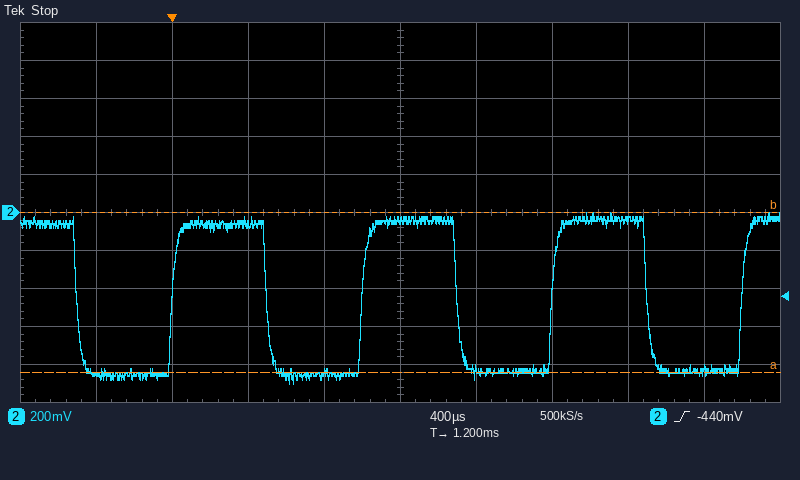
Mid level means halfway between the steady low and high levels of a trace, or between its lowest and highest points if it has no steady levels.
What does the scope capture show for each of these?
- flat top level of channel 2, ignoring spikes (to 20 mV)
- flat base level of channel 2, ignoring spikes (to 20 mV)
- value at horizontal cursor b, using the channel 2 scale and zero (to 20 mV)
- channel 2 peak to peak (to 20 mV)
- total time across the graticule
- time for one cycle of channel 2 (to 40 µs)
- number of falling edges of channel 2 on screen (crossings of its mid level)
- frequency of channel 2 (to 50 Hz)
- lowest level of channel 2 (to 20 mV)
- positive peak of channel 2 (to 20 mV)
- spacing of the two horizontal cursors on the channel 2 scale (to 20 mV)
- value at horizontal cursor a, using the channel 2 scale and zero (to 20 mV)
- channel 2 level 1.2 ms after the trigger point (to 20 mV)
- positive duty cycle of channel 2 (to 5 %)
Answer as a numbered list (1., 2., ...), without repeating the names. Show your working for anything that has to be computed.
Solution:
1. -40 mV
2. -840 mV
3. 0 mV
4. 0 mV − (-900 mV) = 900 mV
5. 4 ms
6. 1.00 ms
7. 4
8. 1 / 1.00 ms ≈ 1.00 kHz
9. -900 mV
10. 0 mV
11. 840 mV
12. -840 mV
13. -40 mV
14. 50 %
